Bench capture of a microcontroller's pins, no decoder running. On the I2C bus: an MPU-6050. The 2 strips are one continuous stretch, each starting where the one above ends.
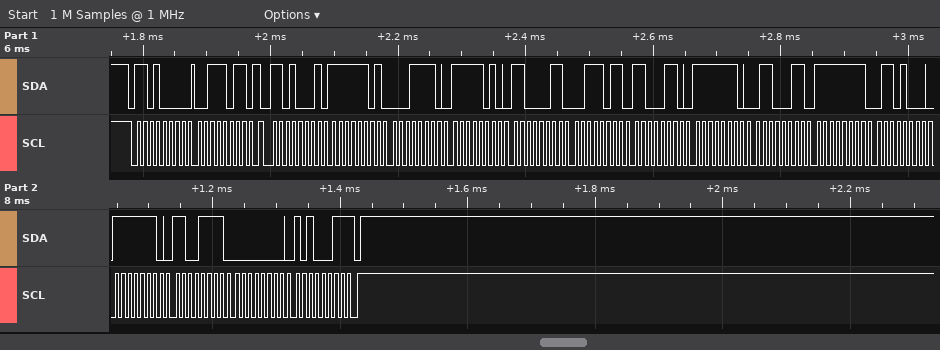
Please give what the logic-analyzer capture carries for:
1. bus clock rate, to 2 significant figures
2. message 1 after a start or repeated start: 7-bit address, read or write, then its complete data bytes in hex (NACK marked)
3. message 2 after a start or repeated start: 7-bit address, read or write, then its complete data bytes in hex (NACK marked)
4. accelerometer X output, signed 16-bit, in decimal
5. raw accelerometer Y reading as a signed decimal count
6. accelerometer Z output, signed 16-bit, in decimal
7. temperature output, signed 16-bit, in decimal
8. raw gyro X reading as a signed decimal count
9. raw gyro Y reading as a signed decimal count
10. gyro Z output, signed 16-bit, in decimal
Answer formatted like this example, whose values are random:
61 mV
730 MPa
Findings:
100 kHz
0x68 write: 3B
0x68 read: FD 1E FA C3 3B C6 FE 63 FF 68 FE CF 00 A3 NACK
-738
-1341
15302
-413
-152
-305
163
